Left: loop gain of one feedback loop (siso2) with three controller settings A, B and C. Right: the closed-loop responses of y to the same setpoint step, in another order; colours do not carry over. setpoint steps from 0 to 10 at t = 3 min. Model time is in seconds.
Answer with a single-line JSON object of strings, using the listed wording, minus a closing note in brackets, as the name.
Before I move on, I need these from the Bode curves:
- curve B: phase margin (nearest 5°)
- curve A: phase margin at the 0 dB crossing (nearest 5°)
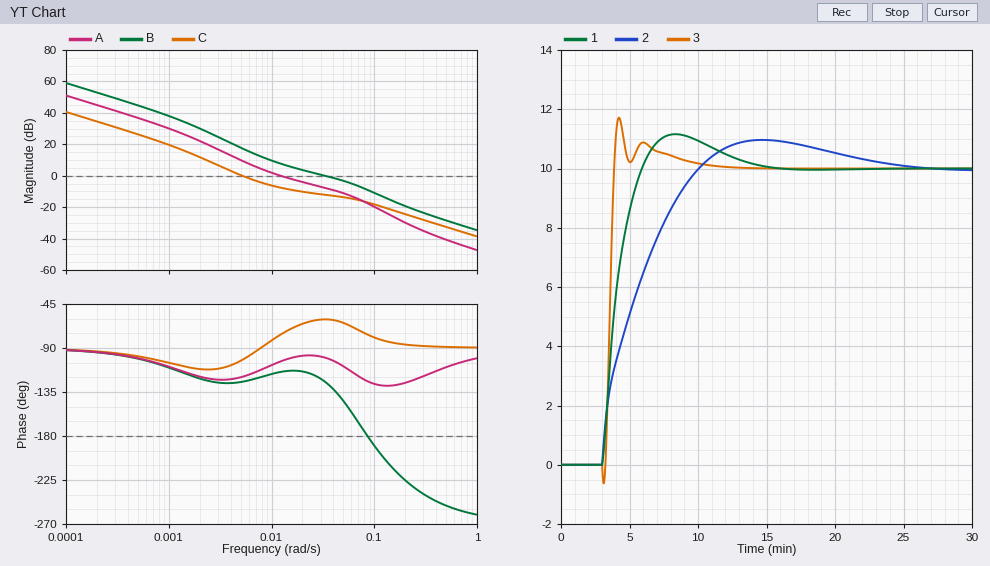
{"curve B: phase margin": "55°", "curve A: phase margin at the 0 dB crossing": "75°"}
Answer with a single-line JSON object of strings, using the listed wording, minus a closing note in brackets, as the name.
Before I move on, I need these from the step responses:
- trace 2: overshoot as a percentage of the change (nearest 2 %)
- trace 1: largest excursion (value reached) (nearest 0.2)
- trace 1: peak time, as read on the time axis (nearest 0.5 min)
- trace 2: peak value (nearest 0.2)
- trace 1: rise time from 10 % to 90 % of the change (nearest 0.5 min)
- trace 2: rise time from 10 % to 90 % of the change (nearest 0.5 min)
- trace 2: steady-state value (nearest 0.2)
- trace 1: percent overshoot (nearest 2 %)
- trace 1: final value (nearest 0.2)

{"trace 2: overshoot as a percentage of the change": "10 %", "trace 1: largest excursion (value reached)": "11.2", "trace 1: peak time, as read on the time axis": "8.5 min", "trace 2: peak value": "11.0", "trace 1: rise time from 10 % to 90 % of the change": "2.0 min", "trace 2: rise time from 10 % to 90 % of the change": "5.5 min", "trace 2: steady-state value": "10.0", "trace 1: percent overshoot": "12 %", "trace 1: final value": "10.0"}
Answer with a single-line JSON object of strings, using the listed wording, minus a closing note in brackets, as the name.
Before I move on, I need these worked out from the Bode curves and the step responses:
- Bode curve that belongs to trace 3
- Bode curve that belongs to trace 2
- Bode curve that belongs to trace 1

{"Bode curve that belongs to trace 3": "B", "Bode curve that belongs to trace 2": "C", "Bode curve that belongs to trace 1": "A"}
